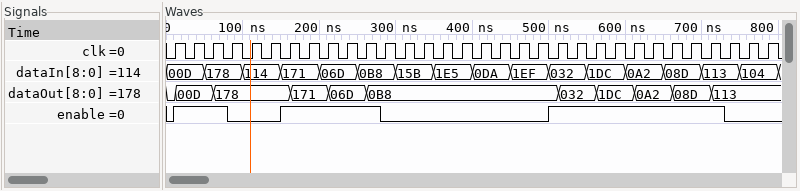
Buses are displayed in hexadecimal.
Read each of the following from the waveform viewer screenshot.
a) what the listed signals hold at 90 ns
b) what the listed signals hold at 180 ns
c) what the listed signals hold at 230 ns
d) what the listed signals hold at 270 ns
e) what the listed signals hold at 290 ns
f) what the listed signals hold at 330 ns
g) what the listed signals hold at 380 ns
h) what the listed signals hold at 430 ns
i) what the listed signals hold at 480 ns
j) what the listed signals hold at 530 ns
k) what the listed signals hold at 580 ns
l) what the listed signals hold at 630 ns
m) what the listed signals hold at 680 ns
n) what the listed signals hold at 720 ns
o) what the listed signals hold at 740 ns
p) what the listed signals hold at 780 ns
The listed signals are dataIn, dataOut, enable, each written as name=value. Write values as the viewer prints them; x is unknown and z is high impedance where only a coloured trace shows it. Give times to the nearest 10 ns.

dataIn=178, dataOut=178, enable=0
dataIn=171, dataOut=171, enable=1
dataIn=06D, dataOut=06D, enable=1
dataIn=0B8, dataOut=0B8, enable=1
dataIn=0B8, dataOut=0B8, enable=0
dataIn=15B, dataOut=0B8, enable=0
dataIn=1E5, dataOut=0B8, enable=0
dataIn=0DA, dataOut=0B8, enable=0
dataIn=1EF, dataOut=0B8, enable=0
dataIn=032, dataOut=032, enable=1
dataIn=1DC, dataOut=1DC, enable=1
dataIn=0A2, dataOut=0A2, enable=1
dataIn=08D, dataOut=08D, enable=1
dataIn=113, dataOut=113, enable=1
dataIn=113, dataOut=113, enable=0
dataIn=104, dataOut=113, enable=0
